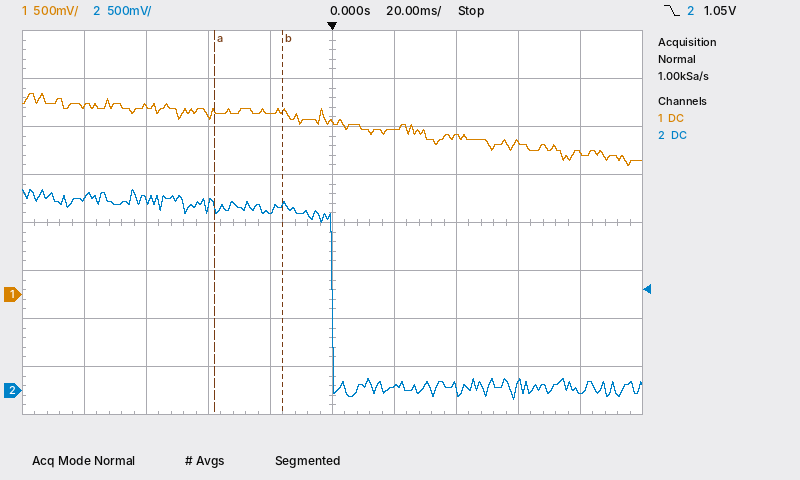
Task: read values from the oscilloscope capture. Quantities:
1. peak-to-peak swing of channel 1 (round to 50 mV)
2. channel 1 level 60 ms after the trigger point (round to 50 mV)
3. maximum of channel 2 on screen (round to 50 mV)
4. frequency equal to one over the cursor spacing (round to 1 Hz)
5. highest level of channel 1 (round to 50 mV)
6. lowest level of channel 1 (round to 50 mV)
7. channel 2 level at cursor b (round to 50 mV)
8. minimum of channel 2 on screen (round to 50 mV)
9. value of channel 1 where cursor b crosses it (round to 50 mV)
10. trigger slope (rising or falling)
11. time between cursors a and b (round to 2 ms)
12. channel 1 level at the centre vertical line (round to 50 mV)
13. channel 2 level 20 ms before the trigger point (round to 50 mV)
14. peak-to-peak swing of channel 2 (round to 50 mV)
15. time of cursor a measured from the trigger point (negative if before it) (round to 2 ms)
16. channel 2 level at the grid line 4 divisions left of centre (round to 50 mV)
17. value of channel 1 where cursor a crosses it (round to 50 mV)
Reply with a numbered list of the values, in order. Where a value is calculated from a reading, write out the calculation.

1. 2.10 V − (1.35 V) = 750 mV
2. 1.60 V
3. 2.10 V
4. 1 / 22 ms ≈ 45 Hz
5. 2.10 V
6. 1.35 V
7. 1.95 V
8. -100 mV
9. 1.90 V
10. falling
11. 22 ms
12. 1.80 V
13. 1.85 V
14. 2.10 V − (-100 mV) = 2.20 V
15. -38 ms
16. 2.00 V
17. 1.90 V
